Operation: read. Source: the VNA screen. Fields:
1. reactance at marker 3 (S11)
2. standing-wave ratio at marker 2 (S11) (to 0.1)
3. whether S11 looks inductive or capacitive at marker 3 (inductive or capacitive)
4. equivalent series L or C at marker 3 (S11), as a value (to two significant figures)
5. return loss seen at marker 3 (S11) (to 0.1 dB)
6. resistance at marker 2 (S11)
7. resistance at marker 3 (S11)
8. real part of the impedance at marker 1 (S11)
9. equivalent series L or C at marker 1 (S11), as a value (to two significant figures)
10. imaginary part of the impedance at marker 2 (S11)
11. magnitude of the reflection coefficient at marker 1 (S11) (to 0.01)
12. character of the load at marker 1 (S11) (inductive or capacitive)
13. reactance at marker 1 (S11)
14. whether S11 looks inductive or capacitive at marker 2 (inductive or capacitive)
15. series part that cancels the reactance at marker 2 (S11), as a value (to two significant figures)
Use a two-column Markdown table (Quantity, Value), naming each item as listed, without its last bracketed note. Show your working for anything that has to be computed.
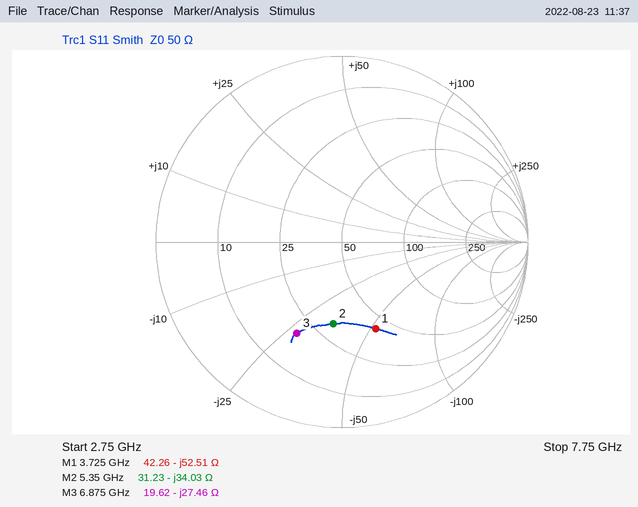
| Quantity | Value |
|---|---|
| reactance at marker 3 | -27.46 Ω |
| standing-wave ratio at marker 2 (S11) | 2.6 |
| whether S11 looks inductive or capacitive at marker 3 | capacitive |
| equivalent series L or C at marker 3 (S11), as a value | C = 1/(2π × 6.875 GHz × 27.46 Ω) ≈ 843 fF, so 840 fF to two significant figures |
| return loss seen at marker 3 (S11) | 5.2 dB |
| resistance at marker 2 | 31.23 Ω |
| resistance at marker 3 | 19.62 Ω |
| real part of the impedance at marker 1 | 42.26 Ω |
| equivalent series L or C at marker 1 (S11), as a value | C = 1/(2π × 3.725 GHz × 52.51 Ω) ≈ 814 fF, so 810 fF to two significant figures |
| imaginary part of the impedance at marker 2 | -34.03 Ω |
| magnitude of the reflection coefficient at marker 1 (S11) | 0.50 |
| character of the load at marker 1 (S11) | capacitive |
| reactance at marker 1 | -52.51 Ω |
| whether S11 looks inductive or capacitive at marker 2 | capacitive |
| series part that cancels the reactance at marker 2 (S11), as a value | L = 34.03 Ω/(2π × 5.35 GHz) ≈ 1.0 nH |
